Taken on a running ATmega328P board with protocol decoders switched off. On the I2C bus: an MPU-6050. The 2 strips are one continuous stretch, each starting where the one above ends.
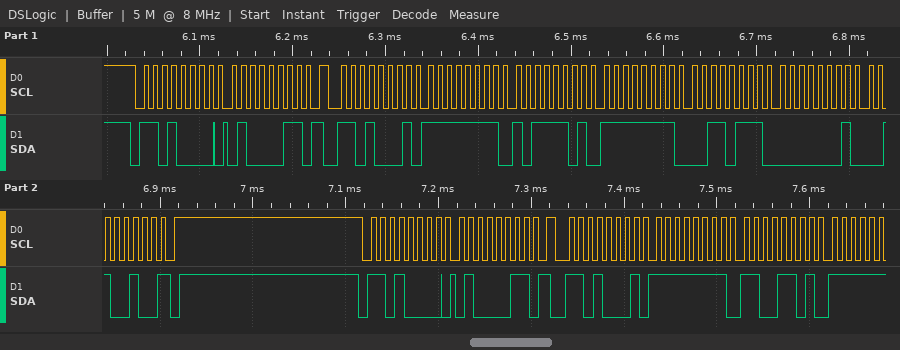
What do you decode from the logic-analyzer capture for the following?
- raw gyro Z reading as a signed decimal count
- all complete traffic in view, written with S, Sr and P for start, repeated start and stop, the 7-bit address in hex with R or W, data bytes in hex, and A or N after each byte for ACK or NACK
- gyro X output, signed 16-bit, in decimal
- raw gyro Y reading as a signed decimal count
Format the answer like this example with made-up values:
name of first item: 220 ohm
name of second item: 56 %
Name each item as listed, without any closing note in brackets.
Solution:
raw gyro Z reading as a signed decimal count: 292
all complete traffic in view, written with S, Sr and P for start, repeated start and stop, the 7-bit address in hex with R or W, data bytes in hex, and A or N after each byte for ACK or NACK: S 68W A 43 A Sr 68R A FF A BD A FF A 37 A 01 A 24 N P S 68W A 43 A Sr 68R A FF A CD A
gyro X output, signed 16-bit, in decimal: -67
raw gyro Y reading as a signed decimal count: -201
